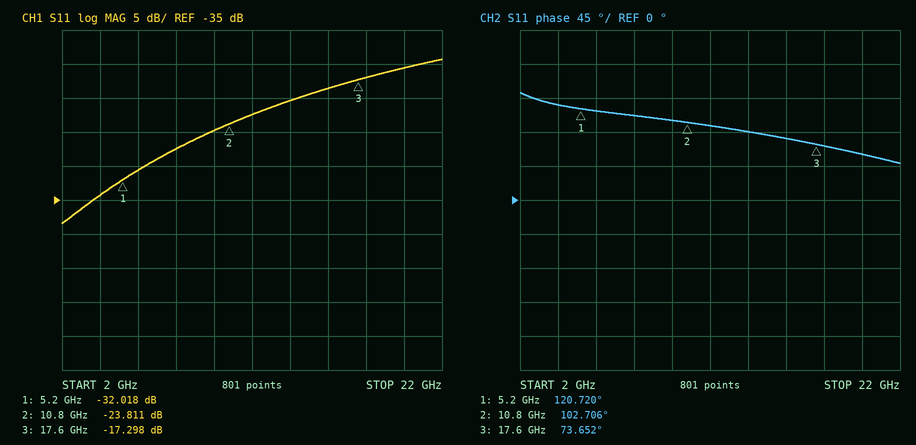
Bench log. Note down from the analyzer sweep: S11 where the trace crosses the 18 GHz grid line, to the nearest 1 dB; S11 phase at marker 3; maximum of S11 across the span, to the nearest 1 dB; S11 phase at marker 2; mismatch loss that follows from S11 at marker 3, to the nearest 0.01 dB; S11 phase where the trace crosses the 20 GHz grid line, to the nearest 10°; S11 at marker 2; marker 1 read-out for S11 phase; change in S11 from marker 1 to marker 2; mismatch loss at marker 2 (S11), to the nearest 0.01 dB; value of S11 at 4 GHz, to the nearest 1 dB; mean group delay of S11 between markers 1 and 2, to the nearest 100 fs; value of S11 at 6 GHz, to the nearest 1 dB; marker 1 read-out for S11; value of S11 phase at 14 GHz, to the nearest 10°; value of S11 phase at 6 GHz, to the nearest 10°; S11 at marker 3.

-17 dB
73.652°
-14 dB
102.706°
0.08 dB
60°
-23.811 dB
120.720°
8.207 dB
0.02 dB
-34 dB
8.9 ps
-31 dB
-32.018 dB
90°
120°
-17.298 dB
